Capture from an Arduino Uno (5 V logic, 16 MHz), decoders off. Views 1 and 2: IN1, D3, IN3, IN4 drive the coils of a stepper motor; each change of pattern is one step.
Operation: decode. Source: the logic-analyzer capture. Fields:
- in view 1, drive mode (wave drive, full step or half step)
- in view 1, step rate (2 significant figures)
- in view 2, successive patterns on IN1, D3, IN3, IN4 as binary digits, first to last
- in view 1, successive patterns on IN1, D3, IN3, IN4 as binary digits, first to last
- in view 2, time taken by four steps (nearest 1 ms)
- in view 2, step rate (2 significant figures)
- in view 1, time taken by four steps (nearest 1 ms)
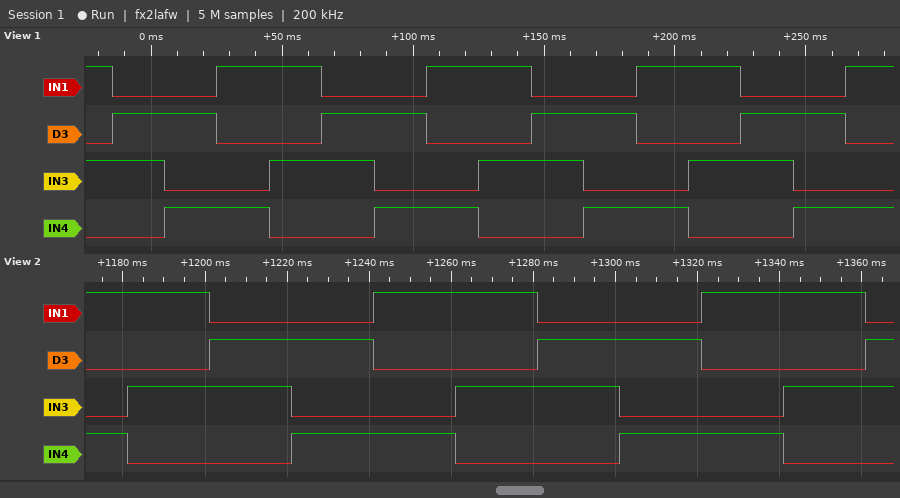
full step
50 steps/s
1001 1010 0110 0101 1001 1010 0110 0101 1001 1010 0110
1010 0110 0101 1001 1010 0110 0101 1001 1010 0110 0101 1001 1010 0110 0101 1001
80 ms
50 steps/s
80 ms
